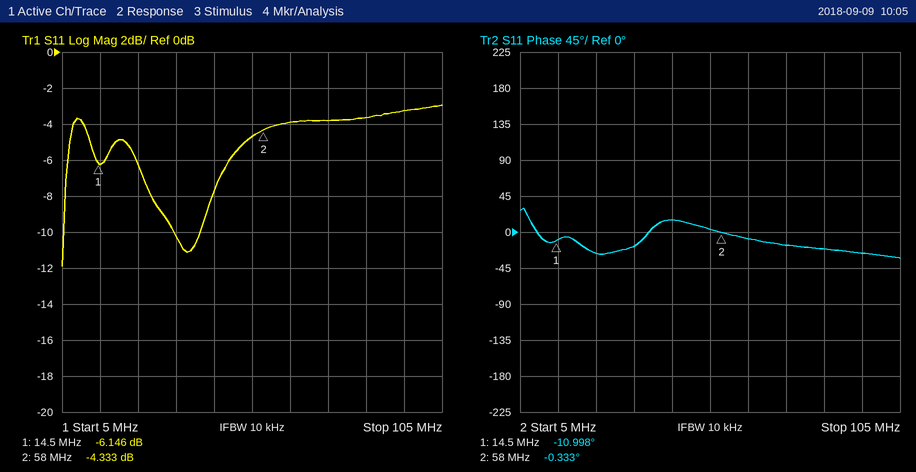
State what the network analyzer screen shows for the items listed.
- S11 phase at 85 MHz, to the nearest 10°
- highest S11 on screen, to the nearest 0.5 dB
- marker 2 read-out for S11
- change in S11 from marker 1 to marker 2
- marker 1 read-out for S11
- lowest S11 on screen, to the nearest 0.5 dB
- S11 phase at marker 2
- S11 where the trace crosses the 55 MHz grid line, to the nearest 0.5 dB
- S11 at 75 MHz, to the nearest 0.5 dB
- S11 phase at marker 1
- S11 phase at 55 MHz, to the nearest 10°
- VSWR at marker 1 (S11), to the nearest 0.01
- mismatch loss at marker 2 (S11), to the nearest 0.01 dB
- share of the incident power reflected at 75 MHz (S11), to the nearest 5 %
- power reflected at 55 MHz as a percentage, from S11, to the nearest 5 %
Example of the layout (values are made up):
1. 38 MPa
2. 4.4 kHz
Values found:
1. -20°
2. -3.0 dB
3. -4.333 dB
4. 1.813 dB
5. -6.146 dB
6. -12.0 dB
7. -0.333°
8. -4.5 dB
9. -4.0 dB
10. -10.998°
11. 0°
12. 2.94
13. 2.00 dB
14. 40 %
15. 35 %
